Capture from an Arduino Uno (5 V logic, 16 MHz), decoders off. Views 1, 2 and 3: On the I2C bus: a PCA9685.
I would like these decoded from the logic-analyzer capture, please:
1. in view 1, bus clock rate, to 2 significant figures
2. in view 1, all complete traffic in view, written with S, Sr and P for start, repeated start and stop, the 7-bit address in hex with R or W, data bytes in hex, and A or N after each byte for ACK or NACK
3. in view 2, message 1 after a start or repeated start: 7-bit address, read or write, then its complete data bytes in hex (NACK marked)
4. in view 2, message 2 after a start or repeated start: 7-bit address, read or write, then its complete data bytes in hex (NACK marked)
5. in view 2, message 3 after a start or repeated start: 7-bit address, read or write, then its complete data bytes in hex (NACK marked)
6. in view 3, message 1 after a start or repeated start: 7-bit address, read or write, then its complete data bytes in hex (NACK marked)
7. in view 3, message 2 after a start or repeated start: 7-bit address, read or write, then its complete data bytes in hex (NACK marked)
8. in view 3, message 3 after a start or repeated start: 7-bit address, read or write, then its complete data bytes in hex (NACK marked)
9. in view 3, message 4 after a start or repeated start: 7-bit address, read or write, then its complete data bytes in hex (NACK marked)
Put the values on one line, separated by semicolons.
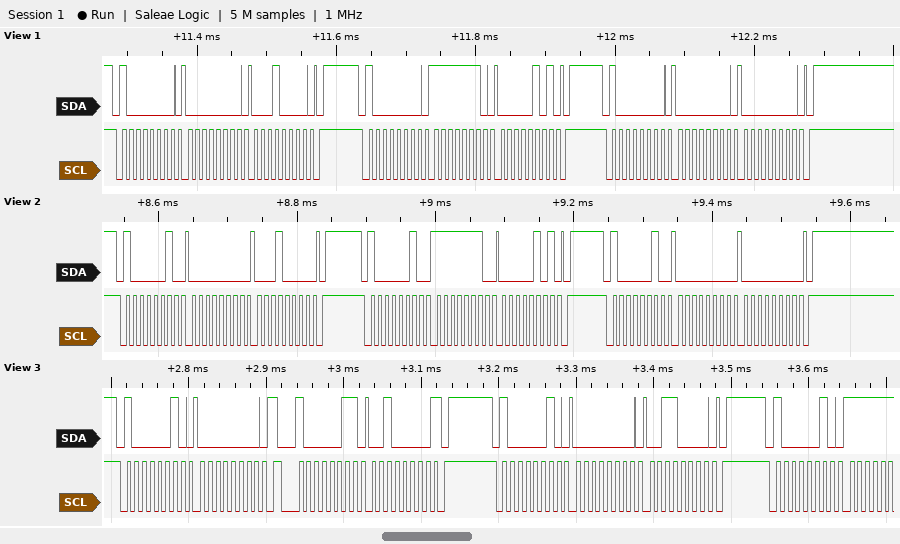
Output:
100 kHz; S 40W A 00 A 10 A P S 40W A FE A 05 A P S 40W A 00 A 00 A P; 0x41 write: 00 10; 0x41 write: FE 05; 0x41 write: 00 00; 0x41 write: 00; 0x41 read: 20 NACK; 0x41 write: 00 30; 0x41 write
